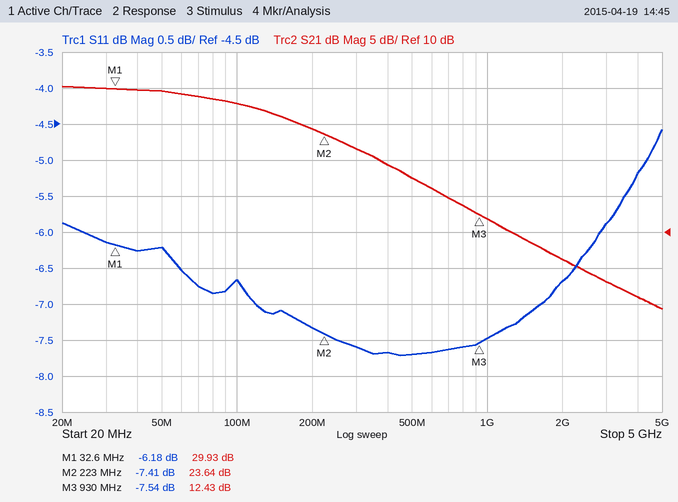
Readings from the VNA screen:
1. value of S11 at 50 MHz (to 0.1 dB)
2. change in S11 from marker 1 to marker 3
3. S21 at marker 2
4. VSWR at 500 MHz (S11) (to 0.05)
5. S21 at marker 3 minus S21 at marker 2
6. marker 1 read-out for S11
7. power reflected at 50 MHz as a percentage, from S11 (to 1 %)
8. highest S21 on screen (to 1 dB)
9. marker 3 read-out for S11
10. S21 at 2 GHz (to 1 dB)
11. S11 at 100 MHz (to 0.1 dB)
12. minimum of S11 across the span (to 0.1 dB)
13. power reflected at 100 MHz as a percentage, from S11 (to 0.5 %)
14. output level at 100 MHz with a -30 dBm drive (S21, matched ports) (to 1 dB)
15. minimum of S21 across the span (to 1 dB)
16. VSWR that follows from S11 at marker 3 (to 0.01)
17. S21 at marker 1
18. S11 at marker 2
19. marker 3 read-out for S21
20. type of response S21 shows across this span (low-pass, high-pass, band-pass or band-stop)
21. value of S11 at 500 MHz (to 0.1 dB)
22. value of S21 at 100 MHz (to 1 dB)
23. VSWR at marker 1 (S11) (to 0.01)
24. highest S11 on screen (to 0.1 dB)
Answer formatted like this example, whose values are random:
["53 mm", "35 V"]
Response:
["-6.2 dB", "-1.36 dB", "23.64 dB", "2.40", "-11.21 dB", "-6.18 dB", "24 %", "30 dB", "-7.54 dB", "6 dB", "-6.7 dB", "-7.7 dB", "21.5 %", "-2 dBm", "-1 dB", "2.45", "29.93 dB", "-7.41 dB", "12.43 dB", "low-pass", "-7.7 dB", "28 dB", "2.93", "-4.6 dB"]
